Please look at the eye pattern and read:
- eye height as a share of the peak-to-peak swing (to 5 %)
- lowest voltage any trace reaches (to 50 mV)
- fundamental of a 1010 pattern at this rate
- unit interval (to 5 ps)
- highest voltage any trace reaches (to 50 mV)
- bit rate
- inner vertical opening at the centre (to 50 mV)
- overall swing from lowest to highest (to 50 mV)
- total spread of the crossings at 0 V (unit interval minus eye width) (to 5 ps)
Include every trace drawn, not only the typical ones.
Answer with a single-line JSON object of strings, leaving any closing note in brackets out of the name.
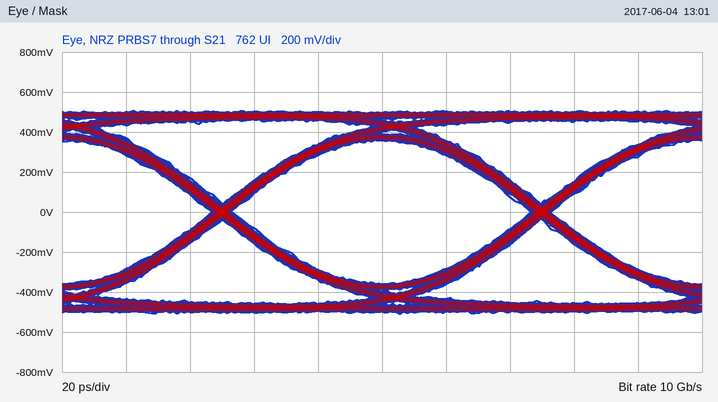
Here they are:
{"eye height as a share of the peak-to-peak swing": "70 %", "lowest voltage any trace reaches": "-500 mV", "fundamental of a 1010 pattern at this rate": "5 GHz", "unit interval": "100 ps", "highest voltage any trace reaches": "500 mV", "bit rate": "10 Gb/s", "inner vertical opening at the centre": "700 mV", "overall swing from lowest to highest": "1.00 V", "total spread of the crossings at 0 V (unit interval minus eye width)": "5 ps"}
